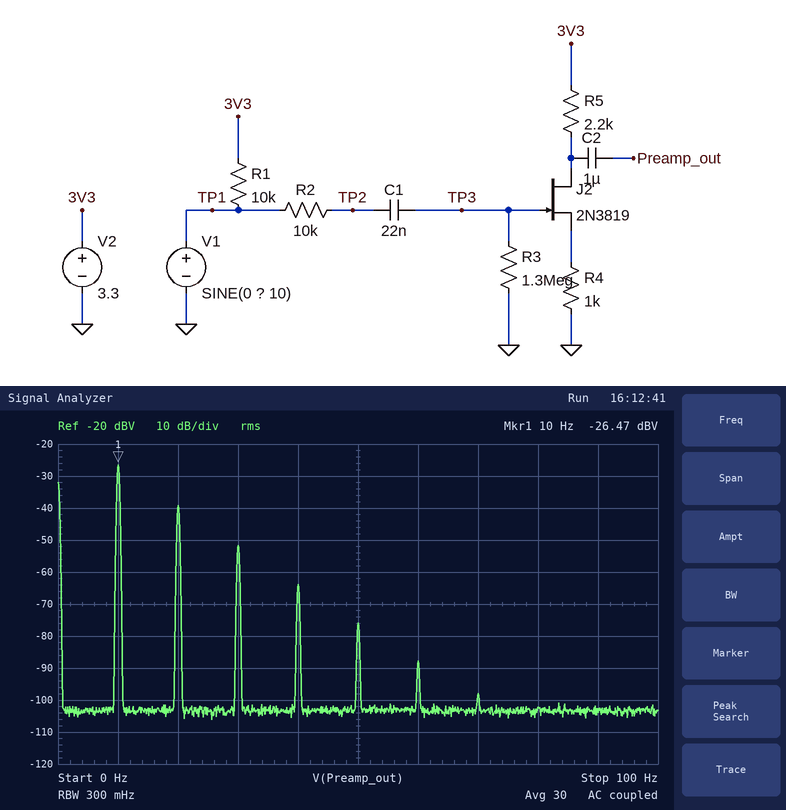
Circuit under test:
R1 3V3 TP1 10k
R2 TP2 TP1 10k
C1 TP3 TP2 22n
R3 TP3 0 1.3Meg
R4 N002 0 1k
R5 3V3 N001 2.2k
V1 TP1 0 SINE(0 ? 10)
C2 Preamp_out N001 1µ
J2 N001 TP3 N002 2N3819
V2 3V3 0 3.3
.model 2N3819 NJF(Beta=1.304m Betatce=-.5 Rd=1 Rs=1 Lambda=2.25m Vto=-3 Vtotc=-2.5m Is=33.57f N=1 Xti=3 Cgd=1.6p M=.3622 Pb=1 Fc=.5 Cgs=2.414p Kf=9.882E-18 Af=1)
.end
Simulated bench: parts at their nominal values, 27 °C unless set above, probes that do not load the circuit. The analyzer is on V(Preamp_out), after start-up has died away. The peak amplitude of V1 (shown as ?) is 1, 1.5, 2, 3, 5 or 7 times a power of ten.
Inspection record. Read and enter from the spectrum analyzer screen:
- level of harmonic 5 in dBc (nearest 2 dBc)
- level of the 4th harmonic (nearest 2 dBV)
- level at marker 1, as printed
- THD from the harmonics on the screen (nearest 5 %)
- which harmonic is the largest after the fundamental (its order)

-50 dBc
-64 dBV
-26.47 dBV
25 %
2
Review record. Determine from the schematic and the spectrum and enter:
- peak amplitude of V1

1 V
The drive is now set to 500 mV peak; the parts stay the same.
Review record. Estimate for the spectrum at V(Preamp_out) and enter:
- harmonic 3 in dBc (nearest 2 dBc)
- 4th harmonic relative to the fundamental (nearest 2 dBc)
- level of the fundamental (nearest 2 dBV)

-38 dBc
-56 dBc
-34 dBV
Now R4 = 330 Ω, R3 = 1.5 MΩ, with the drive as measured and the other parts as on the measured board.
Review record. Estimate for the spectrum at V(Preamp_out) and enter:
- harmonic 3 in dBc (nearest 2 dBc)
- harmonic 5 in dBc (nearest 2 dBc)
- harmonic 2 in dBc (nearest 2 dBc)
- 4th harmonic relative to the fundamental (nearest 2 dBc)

-30 dBc
-58 dBc
-14 dBc
-40 dBc
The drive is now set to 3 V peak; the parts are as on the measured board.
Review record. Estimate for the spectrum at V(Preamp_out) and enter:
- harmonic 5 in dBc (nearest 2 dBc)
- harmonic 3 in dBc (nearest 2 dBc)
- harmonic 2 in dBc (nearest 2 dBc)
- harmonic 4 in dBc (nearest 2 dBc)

-22 dBc
-18 dBc
-6 dBc
-24 dBc
